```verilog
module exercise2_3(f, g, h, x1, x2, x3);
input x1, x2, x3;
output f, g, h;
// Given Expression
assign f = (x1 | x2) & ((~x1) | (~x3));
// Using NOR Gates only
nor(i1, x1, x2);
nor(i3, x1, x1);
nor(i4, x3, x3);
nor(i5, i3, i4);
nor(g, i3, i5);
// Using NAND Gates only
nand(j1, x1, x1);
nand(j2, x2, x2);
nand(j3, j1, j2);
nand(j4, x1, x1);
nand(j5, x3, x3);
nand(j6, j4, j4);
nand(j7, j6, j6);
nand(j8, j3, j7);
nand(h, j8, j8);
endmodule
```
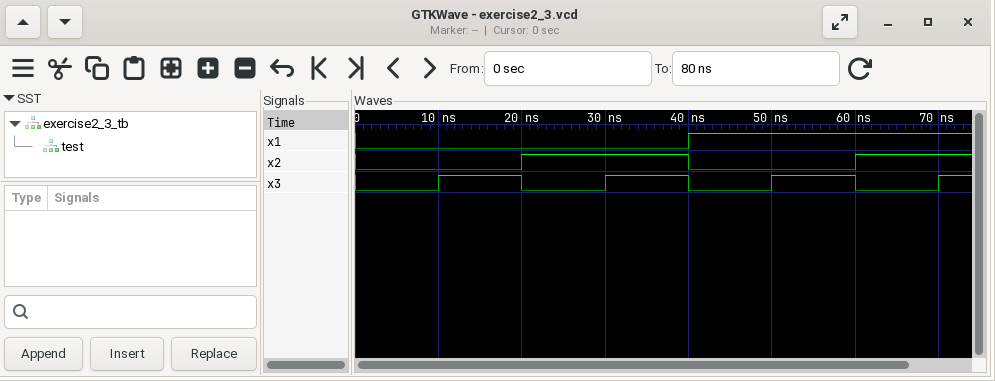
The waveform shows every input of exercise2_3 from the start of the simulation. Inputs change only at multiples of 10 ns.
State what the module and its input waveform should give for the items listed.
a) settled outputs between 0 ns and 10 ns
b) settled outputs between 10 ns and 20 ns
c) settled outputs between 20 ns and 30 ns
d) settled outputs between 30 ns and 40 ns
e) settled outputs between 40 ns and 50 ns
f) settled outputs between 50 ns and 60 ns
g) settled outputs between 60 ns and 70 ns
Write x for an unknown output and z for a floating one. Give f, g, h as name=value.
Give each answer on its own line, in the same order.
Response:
f=0, g=0, h=0
f=0, g=0, h=0
f=1, g=0, h=1
f=1, g=0, h=1
f=1, g=1, h=0
f=0, g=0, h=0
f=1, g=1, h=0
